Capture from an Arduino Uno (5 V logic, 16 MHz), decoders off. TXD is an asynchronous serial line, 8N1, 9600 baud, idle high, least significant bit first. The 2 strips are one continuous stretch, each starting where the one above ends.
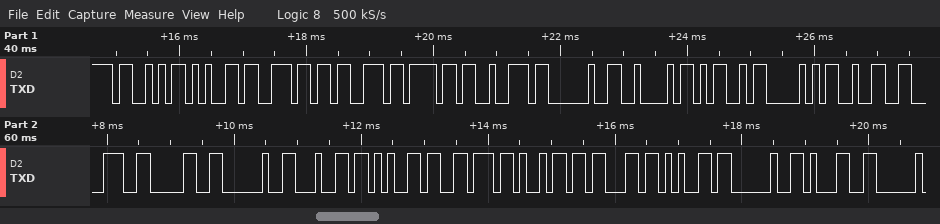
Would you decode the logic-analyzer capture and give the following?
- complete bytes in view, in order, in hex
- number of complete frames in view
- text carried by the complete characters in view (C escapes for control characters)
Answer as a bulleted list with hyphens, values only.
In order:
- 53 65 6E 73 6F 72 20 42 4D 50 32 38 30 20 64 65 76 69 63 65 20 31
- 22
- "Sensor BMP280 device 1"
